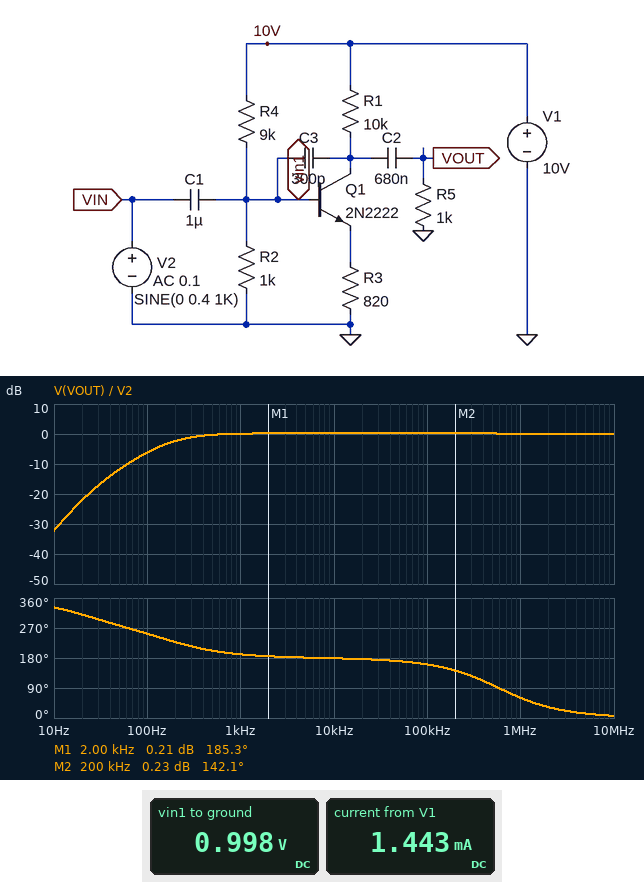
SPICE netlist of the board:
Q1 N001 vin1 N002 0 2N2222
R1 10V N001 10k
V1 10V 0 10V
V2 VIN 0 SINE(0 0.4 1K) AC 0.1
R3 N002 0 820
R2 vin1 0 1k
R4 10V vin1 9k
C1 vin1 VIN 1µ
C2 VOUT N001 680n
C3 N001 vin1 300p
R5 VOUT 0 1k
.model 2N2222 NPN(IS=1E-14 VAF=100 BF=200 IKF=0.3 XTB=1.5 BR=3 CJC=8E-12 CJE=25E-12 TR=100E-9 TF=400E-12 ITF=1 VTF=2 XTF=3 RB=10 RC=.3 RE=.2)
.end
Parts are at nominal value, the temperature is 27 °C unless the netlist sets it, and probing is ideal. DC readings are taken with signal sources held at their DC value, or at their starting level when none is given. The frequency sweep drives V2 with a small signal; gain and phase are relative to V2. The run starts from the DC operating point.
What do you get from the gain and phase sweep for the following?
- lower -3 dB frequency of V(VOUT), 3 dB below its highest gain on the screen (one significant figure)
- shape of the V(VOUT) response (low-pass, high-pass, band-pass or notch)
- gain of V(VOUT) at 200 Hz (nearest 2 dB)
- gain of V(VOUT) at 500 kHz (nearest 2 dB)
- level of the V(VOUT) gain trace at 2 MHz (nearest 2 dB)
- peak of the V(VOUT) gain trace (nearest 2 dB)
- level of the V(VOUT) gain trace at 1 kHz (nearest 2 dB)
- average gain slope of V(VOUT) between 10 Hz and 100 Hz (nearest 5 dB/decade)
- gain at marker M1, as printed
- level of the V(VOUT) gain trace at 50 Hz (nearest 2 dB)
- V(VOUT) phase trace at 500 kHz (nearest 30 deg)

200 Hz
high-pass
-2 dB
0 dB
0 dB
0 dB
0 dB
25 dB/decade
0.21 dB
-12 dB
90 deg
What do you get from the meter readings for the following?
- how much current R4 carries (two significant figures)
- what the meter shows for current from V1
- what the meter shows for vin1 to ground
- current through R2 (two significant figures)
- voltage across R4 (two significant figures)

1.0 mA
1.443 mA
0.998 V
1.0 mA
9.0 V
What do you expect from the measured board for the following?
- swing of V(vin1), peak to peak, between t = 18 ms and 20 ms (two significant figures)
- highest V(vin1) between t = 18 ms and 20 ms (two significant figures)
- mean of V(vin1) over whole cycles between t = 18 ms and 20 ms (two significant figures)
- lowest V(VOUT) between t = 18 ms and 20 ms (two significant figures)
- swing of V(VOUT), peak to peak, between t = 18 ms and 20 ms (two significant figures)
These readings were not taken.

790 mV
1.4 V
1.0 V
-400 mV
780 mV
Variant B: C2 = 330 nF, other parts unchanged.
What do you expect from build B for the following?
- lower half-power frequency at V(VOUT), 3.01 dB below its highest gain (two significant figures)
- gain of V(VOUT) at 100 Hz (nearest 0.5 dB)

190 Hz
-6.5 dB
